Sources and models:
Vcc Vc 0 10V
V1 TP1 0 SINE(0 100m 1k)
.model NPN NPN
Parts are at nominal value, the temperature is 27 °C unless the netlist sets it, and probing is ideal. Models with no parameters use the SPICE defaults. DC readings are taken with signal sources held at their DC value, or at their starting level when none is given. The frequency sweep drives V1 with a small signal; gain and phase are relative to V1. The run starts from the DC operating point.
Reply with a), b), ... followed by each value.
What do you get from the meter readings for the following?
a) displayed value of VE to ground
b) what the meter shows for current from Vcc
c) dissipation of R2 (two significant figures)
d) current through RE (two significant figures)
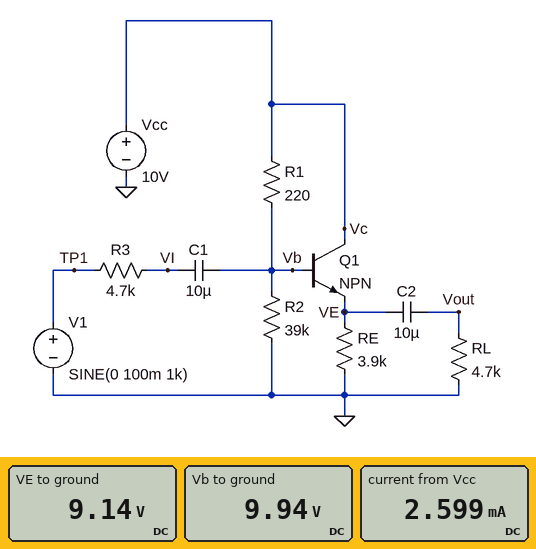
a) 9.14 V
b) 2.599 mA
c) 2.5 mW
d) 2.3 mA
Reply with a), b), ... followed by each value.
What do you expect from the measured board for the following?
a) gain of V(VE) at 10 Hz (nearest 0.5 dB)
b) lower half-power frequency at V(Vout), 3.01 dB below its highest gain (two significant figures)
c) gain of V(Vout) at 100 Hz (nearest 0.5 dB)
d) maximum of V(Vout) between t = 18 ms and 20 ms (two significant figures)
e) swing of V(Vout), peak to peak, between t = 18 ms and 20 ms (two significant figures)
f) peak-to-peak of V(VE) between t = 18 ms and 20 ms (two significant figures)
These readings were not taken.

a) -27.5 dB
b) 5.1 Hz
c) -27.0 dB
d) 4.4 mV
e) 8.8 mV
f) 8.8 mV
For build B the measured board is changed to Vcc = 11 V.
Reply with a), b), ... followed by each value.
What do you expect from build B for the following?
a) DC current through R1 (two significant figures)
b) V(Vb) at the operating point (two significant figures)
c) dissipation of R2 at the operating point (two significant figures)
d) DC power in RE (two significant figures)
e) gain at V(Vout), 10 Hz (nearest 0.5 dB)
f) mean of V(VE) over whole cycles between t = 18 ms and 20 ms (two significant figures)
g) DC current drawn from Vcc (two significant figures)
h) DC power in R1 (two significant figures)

a) 310 µA
b) 11 V
c) 3.1 mW
d) 26 mW
e) -28.0 dB
f) 10 V
g) 2.9 mA
h) 21 µW
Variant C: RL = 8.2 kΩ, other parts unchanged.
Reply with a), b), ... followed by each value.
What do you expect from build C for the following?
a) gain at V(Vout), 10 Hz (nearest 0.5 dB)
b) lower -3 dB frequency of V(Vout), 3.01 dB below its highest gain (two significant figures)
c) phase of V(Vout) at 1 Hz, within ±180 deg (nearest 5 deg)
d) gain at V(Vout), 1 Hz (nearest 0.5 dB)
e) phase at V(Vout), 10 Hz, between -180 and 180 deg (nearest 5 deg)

a) -27.5 dB
b) 4.1 Hz
c) 135 deg
d) -44.5 dB
e) 30 deg
